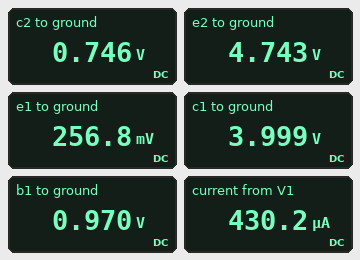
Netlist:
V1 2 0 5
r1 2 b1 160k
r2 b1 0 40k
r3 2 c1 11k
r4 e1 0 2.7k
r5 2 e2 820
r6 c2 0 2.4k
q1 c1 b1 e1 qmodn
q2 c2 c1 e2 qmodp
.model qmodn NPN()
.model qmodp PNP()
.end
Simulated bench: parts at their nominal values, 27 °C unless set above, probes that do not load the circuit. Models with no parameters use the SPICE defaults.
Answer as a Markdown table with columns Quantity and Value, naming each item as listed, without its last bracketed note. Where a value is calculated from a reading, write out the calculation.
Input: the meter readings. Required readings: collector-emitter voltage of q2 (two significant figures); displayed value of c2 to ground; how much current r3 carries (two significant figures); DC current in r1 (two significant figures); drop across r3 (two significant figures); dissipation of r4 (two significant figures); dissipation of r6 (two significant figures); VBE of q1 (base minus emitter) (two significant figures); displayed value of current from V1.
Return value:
| Quantity | Value |
|---|---|
| collector-emitter voltage of q2 | 746 mV - 4.743 V = -4.0 V |
| displayed value of c2 to ground | 0.746 V |
| how much current r3 carries | (5 V - 3.999 V) / 11 kΩ = 91 µA |
| DC current in r1 | (5 V - 970 mV) / 160 kΩ = 25 µA |
| drop across r3 | 5 V - 3.999 V = 1.0 V |
| dissipation of r4 | (256.8 mV)^2 / 2.7 kΩ = 24 µW |
| dissipation of r6 | (746 mV)^2 / 2.4 kΩ = 230 µW |
| VBE of q1 (base minus emitter) | 970 mV - 256.8 mV = 710 mV |
| displayed value of current from V1 | 430.2 µA |
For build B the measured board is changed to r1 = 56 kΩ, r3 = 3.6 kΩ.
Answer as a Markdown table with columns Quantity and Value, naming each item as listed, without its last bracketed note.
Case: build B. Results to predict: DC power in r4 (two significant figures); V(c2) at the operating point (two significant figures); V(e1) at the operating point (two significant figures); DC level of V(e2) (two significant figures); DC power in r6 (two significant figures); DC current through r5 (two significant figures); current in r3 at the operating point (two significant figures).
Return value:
| Quantity | Value |
|---|---|
| DC power in r4 | 560 µW |
| V(c2) at the operating point | 2.3 V |
| V(e1) at the operating point | 1.2 V |
| DC level of V(e2) | 4.2 V |
| DC power in r6 | 2.3 mW |
| DC current through r5 | 990 µA |
| current in r3 at the operating point | 440 µA |
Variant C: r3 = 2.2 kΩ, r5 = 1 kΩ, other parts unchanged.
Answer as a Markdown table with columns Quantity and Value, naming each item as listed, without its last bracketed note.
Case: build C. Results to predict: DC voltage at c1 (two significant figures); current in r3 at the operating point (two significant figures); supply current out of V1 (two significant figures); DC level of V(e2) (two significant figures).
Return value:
| Quantity | Value |
|---|---|
| DC voltage at c1 | 4.8 V |
| current in r3 at the operating point | 94 µA |
| supply current out of V1 | 120 µA |
| DC level of V(e2) | 5.0 V |
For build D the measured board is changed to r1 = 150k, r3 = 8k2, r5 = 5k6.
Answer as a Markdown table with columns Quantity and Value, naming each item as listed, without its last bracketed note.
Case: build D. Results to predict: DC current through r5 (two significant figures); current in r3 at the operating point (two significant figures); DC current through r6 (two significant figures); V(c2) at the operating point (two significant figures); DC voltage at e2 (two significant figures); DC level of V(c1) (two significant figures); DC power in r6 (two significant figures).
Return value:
| Quantity | Value |
|---|---|
| DC current through r5 | 38 µA |
| current in r3 at the operating point | 110 µA |
| DC current through r6 | 37 µA |
| V(c2) at the operating point | 90 mV |
| DC voltage at e2 | 4.8 V |
| DC level of V(c1) | 4.1 V |
| DC power in r6 | 3.4 µW |
